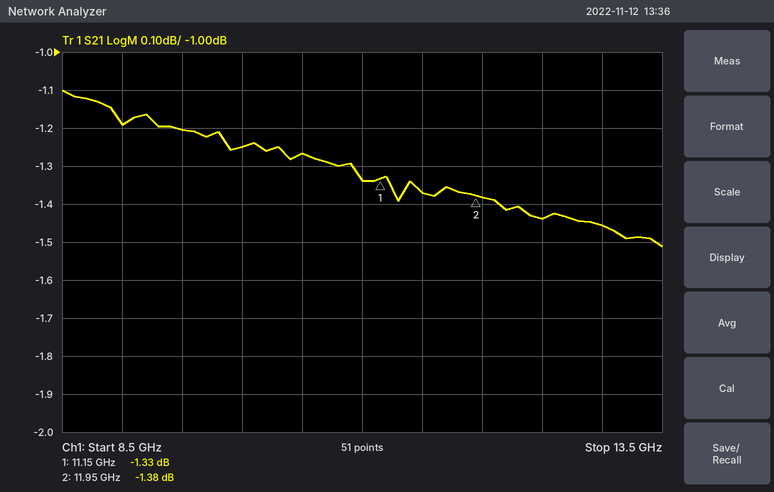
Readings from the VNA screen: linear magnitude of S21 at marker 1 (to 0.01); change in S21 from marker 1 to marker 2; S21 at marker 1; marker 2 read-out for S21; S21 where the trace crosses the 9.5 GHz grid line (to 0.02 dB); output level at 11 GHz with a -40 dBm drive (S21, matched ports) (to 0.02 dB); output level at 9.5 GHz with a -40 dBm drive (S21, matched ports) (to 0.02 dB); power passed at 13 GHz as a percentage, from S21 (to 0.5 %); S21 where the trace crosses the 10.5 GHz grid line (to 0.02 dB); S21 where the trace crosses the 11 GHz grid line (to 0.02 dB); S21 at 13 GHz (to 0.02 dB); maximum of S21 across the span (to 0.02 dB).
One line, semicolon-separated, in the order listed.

0.86; -0.05 dB; -1.33 dB; -1.38 dB; -1.20 dB; -41.34 dBm; -41.20 dBm; 71.5 %; -1.26 dB; -1.34 dB; -1.46 dB; -1.10 dB
